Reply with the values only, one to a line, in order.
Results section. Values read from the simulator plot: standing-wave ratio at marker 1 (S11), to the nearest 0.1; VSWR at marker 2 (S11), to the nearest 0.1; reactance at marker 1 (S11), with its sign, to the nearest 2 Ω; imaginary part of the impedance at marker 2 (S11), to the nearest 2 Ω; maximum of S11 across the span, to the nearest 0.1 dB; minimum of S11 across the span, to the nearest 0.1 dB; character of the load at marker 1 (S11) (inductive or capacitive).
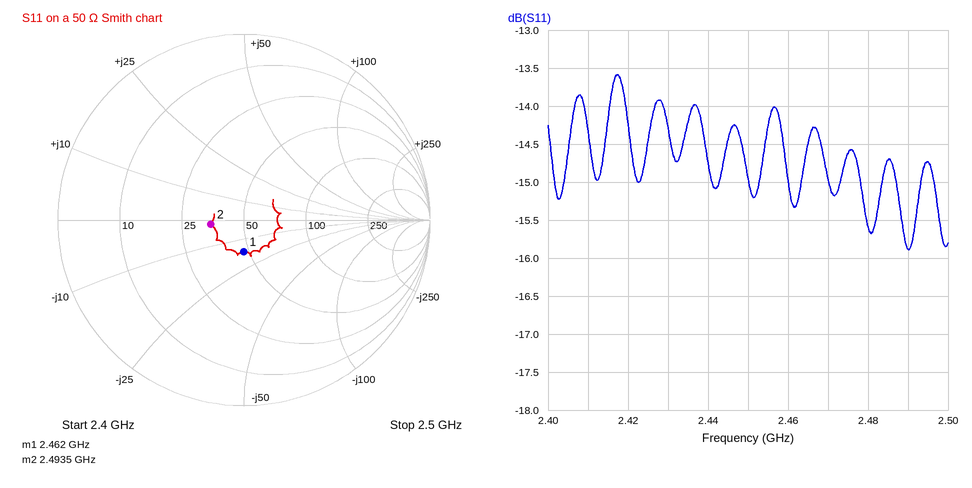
1.4
1.4
-16 Ω
-2 Ω
-13.6 dB
-15.9 dB
capacitive
